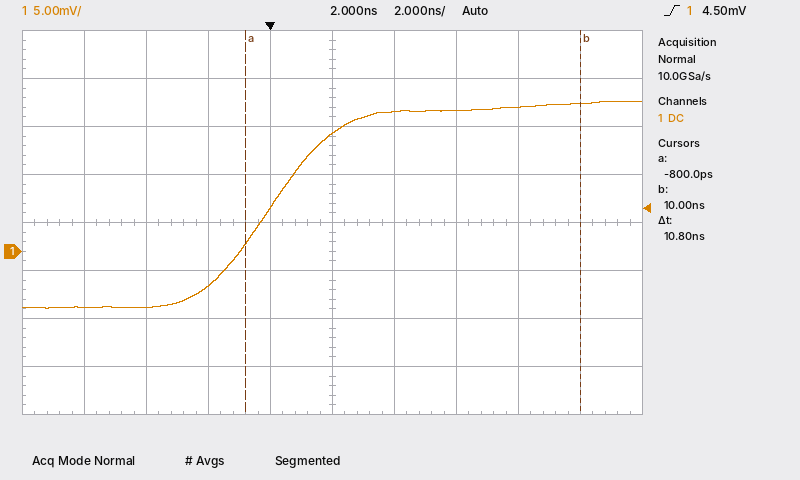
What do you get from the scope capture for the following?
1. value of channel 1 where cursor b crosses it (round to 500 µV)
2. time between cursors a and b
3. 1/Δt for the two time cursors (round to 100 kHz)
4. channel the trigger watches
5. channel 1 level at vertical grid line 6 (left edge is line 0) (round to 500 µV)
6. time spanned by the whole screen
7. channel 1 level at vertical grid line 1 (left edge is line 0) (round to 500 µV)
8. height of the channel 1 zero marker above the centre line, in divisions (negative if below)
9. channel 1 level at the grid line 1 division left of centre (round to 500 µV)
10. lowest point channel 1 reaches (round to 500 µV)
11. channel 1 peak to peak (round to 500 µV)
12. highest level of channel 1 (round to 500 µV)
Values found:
15.5 mV
10.8 ns
92.6 MHz
channel 1
14.5 mV
20 ns
-6.0 mV
-0.6 div
4.5 mV
-6.0 mV
21.5 mV
15.5 mV
